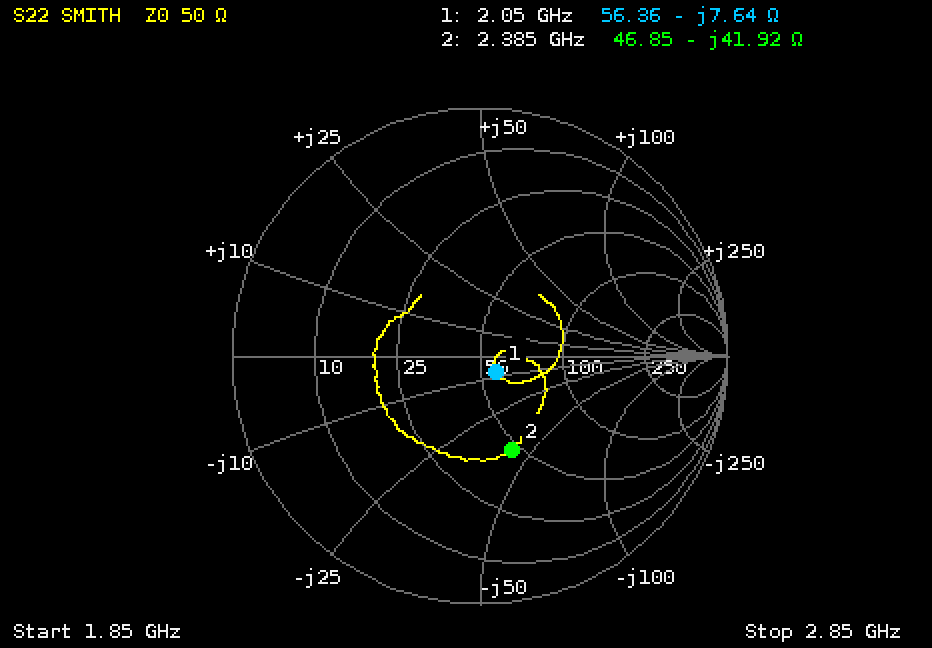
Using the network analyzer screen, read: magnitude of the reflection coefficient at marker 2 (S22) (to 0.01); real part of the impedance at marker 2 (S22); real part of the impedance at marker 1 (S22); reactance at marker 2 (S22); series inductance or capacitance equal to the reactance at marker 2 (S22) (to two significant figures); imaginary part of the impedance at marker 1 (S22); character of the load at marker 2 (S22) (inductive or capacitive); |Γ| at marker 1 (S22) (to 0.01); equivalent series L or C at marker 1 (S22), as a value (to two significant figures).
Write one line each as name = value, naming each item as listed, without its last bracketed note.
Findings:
magnitude of the reflection coefficient at marker 2 (S22) = 0.40
real part of the impedance at marker 2 = 46.85 Ω
real part of the impedance at marker 1 = 56.36 Ω
reactance at marker 2 = -41.92 Ω
series inductance or capacitance equal to the reactance at marker 2 (S22) = 1.6 pF
imaginary part of the impedance at marker 1 = -7.64 Ω
character of the load at marker 2 (S22) = capacitive
|Γ| at marker 1 (S22) = 0.09
equivalent series L or C at marker 1 (S22), as a value = 10 pF
